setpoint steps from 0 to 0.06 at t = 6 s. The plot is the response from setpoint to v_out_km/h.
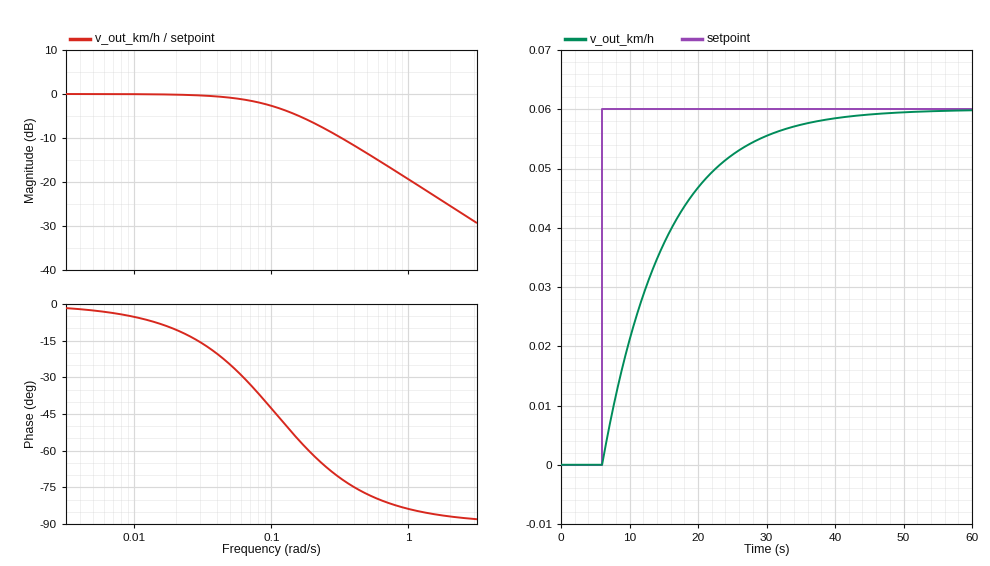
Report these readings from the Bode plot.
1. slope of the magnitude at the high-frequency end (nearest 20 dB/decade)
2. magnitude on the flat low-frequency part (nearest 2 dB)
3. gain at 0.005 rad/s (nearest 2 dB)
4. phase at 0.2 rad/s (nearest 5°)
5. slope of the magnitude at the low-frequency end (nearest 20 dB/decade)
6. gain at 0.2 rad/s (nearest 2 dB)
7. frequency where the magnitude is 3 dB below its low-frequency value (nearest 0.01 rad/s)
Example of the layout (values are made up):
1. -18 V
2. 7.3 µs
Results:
1. -20 dB/decade
2. 0 dB
3. 0 dB
4. -60°
5. 0 dB/decade
6. -6 dB
7. 0.11 rad/s
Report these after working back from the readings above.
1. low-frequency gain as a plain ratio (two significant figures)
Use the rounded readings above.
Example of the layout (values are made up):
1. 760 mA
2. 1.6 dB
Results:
1. 1.0
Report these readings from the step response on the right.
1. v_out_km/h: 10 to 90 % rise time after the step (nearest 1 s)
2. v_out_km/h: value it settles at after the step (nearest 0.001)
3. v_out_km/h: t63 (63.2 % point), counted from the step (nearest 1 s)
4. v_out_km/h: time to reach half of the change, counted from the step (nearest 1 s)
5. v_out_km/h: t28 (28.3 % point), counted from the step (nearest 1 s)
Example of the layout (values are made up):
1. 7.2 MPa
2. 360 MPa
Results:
1. 20 s
2. 0.060
3. 9 s
4. 6 s
5. 3 s
